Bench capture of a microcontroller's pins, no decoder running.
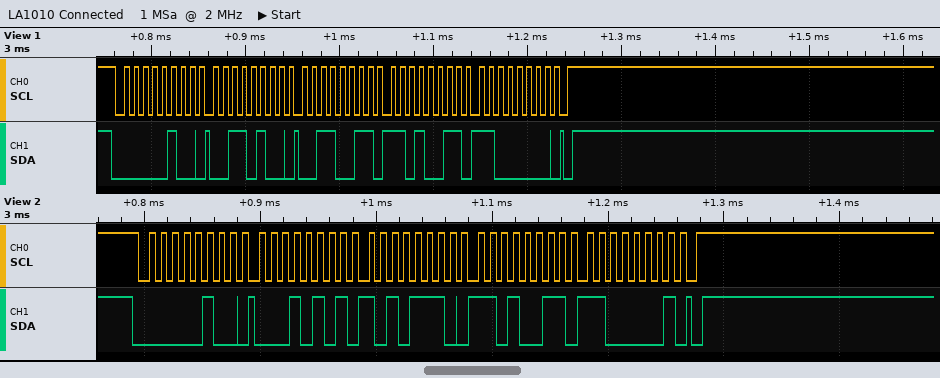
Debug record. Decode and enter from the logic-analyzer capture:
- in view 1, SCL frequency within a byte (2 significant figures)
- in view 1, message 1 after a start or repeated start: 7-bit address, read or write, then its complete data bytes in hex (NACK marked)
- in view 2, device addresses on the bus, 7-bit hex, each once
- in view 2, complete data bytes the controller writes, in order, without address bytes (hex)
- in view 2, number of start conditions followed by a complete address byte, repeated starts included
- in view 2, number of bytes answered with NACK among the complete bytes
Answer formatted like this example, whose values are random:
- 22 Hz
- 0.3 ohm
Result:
- 100 kHz
- 0x02 write: 34 33 D3 C0
- 0x02
- 15 AE D3 C1
- 1
- 0
